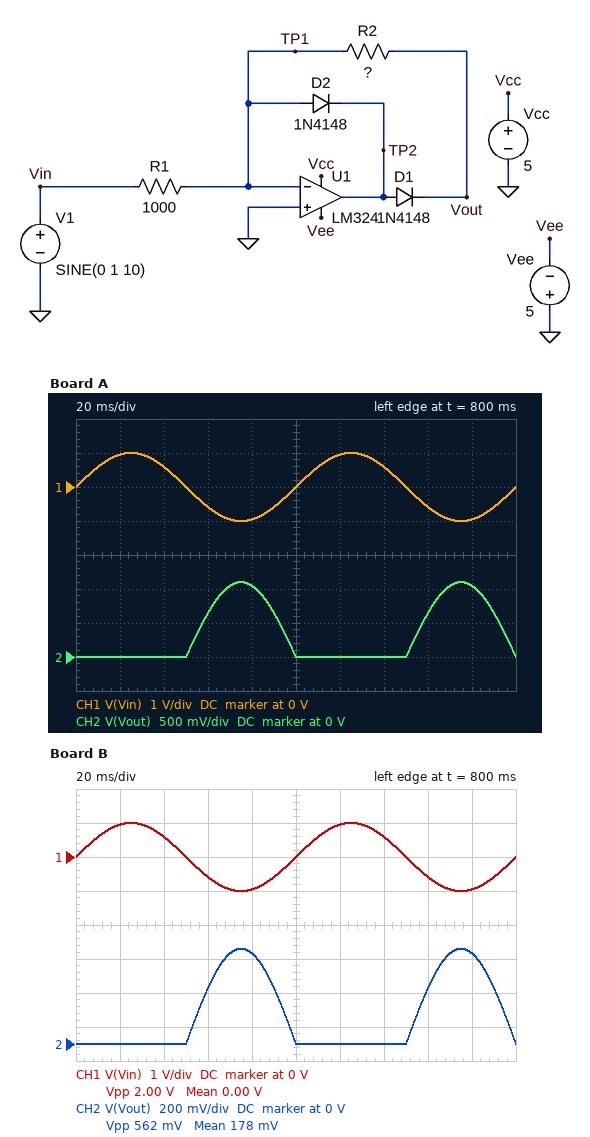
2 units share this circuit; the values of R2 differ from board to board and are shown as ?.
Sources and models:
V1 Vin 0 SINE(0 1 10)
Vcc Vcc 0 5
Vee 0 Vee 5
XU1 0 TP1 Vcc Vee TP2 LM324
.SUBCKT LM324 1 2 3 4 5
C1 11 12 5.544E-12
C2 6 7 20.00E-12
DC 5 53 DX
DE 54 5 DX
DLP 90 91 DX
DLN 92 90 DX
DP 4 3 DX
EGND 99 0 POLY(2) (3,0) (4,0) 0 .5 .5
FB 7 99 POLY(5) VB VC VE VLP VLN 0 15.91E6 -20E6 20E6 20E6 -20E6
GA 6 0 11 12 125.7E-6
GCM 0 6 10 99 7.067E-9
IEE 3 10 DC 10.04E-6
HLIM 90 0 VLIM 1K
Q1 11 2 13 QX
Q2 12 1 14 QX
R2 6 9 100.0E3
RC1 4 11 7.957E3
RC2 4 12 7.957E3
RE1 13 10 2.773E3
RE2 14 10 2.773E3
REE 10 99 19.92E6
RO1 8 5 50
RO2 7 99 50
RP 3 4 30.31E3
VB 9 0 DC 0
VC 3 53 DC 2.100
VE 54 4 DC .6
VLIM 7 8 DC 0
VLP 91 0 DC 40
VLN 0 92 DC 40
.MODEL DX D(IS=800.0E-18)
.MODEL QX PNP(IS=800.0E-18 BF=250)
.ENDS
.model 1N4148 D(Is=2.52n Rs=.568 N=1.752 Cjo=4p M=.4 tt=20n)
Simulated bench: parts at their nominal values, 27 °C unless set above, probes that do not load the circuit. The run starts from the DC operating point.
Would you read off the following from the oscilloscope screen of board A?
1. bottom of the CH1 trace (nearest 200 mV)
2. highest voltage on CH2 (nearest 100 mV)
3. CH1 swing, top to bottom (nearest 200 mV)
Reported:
-1.0 V
1.1 V
2.0 V
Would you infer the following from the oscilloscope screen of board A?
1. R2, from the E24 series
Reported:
1.1 kΩ
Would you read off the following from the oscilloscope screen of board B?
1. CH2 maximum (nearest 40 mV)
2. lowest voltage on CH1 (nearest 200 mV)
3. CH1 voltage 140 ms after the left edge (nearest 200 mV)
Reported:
560 mV
-1.0 V
600 mV
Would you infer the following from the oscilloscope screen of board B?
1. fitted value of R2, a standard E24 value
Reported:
560 Ω
